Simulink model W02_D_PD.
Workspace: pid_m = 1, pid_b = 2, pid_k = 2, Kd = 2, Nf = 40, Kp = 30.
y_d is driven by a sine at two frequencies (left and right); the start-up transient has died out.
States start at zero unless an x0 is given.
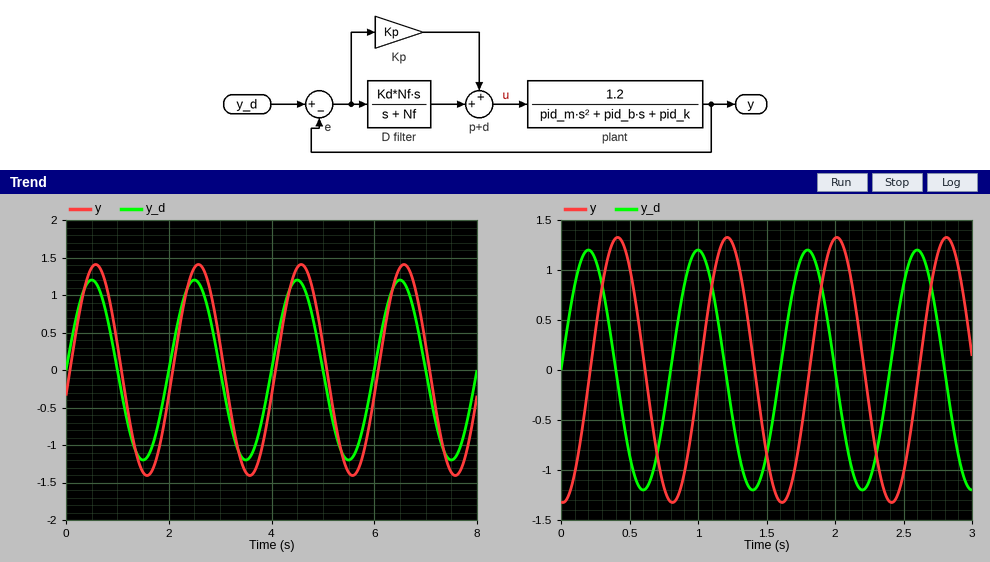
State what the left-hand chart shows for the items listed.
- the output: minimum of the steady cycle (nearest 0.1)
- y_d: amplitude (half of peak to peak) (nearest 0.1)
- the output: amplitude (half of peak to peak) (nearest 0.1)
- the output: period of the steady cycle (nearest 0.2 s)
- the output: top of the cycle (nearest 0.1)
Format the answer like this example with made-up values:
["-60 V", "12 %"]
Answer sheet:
["-1.4", "1.2", "1.4", "2.0 s", "1.4"]
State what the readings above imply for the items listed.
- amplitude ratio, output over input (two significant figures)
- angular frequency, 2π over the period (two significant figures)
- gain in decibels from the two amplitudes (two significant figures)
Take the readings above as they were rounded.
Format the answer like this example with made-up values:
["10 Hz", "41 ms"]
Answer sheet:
["1.2", "3.1 rad/s", "1.3 dB"]
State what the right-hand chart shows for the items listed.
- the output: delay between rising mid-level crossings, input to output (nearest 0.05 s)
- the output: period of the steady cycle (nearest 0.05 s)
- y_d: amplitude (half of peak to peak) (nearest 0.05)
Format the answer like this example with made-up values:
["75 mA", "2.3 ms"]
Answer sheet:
["0.20 s", "0.80 s", "1.20"]
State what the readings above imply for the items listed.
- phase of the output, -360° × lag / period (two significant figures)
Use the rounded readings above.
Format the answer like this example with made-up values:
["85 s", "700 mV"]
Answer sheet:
["-90°"]
